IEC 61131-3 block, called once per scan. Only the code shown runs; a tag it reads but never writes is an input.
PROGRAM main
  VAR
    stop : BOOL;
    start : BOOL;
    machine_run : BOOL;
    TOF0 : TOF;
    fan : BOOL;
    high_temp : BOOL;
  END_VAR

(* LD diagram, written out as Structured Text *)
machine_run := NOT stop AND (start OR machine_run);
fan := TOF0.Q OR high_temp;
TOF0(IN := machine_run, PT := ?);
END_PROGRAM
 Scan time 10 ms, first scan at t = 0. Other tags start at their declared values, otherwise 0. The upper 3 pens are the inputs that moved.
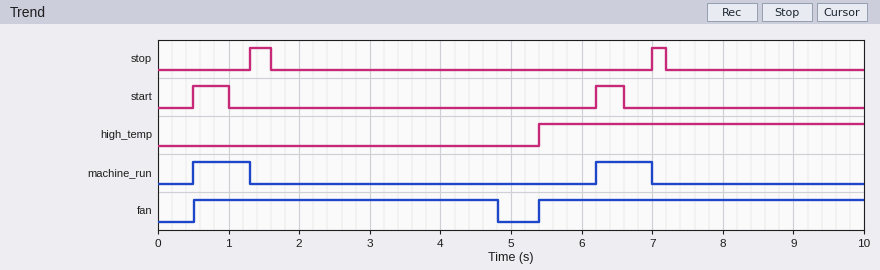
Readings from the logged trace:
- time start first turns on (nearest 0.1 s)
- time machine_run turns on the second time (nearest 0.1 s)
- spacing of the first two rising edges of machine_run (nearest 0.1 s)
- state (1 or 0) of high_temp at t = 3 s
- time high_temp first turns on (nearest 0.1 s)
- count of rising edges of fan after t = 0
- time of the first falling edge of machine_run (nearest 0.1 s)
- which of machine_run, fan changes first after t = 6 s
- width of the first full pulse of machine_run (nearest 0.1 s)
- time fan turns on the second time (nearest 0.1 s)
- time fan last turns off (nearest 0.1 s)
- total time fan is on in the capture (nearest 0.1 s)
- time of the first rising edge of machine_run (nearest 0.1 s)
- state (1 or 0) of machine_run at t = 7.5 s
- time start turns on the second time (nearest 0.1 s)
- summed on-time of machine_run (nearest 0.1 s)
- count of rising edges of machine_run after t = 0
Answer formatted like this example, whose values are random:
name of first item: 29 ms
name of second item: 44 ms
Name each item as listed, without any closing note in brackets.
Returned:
time start first turns on: 0.5 s
time machine_run turns on the second time: 6.2 s
spacing of the first two rising edges of machine_run: 5.7 s
state (1 or 0) of high_temp at t = 3 s: 0
time high_temp first turns on: 5.4 s
count of rising edges of fan after t = 0: 2
time of the first falling edge of machine_run: 1.3 s
which of machine_run, fan changes first after t = 6 s: machine_run
width of the first full pulse of machine_run: 0.8 s
time fan turns on the second time: 5.4 s
time fan last turns off: 4.8 s
total time fan is on in the capture: 8.9 s
time of the first rising edge of machine_run: 0.5 s
state (1 or 0) of machine_run at t = 7.5 s: 0
time start turns on the second time: 6.2 s
summed on-time of machine_run: 1.6 s
count of rising edges of machine_run after t = 0: 2
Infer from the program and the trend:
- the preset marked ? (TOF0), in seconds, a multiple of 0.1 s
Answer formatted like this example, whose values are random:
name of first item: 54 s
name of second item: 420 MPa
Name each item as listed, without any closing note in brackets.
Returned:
the preset marked ? (TOF0), in seconds, a multiple of 0.1 s: 3.5 s
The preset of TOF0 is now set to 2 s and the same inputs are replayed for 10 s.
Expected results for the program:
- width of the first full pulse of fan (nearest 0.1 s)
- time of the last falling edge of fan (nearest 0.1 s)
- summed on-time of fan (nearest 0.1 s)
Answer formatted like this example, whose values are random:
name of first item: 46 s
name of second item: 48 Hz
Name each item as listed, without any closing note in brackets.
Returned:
width of the first full pulse of fan: 2.8 s
time of the last falling edge of fan: 3.3 s
summed on-time of fan: 7.4 s
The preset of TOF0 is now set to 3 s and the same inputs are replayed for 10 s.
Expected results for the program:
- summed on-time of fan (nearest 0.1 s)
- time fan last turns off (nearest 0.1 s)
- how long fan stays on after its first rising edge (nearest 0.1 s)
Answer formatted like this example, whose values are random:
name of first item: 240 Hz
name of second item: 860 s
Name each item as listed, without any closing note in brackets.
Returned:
summed on-time of fan: 8.4 s
time fan last turns off: 4.3 s
how long fan stays on after its first rising edge: 3.8 s
